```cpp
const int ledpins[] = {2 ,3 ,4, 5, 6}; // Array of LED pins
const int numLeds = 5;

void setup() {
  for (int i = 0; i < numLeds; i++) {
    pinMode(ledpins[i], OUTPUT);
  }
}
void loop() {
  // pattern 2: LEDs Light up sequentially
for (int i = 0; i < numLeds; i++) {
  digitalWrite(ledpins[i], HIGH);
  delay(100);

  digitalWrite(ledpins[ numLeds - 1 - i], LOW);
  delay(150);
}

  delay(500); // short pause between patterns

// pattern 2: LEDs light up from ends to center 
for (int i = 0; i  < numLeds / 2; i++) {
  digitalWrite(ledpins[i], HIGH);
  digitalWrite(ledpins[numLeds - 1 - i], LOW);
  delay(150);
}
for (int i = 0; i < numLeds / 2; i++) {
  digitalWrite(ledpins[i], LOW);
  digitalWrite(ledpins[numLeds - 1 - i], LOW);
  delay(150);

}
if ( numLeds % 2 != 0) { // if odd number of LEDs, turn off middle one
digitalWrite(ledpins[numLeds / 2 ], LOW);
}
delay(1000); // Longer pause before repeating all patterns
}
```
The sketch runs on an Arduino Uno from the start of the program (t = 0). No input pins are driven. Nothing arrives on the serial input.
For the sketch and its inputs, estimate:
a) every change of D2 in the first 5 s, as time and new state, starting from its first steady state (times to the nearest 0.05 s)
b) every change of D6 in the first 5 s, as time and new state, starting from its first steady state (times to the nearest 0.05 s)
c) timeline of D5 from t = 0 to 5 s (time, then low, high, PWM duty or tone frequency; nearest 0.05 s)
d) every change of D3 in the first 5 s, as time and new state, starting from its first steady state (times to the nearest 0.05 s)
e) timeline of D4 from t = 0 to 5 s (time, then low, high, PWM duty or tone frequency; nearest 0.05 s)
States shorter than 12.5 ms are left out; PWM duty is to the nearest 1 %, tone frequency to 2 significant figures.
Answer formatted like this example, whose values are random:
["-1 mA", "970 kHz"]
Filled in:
["0 s high; 1.1 s low; 1.75 s high; 2.05 s low; 3.35 s high; 4.45 s low", "0 s low; 1 s high; 1.75 s low; 4.35 s high", "0 s low; 0.75 s high; 1.9 s low; 4.1 s high", "0 s low; 0.25 s high; 0.85 s low; 1.9 s high; 2.2 s low; 3.6 s high; 4.2 s low", "0 s low; 0.5 s high; 0.6 s low; 3.85 s high; 3.95 s low"]
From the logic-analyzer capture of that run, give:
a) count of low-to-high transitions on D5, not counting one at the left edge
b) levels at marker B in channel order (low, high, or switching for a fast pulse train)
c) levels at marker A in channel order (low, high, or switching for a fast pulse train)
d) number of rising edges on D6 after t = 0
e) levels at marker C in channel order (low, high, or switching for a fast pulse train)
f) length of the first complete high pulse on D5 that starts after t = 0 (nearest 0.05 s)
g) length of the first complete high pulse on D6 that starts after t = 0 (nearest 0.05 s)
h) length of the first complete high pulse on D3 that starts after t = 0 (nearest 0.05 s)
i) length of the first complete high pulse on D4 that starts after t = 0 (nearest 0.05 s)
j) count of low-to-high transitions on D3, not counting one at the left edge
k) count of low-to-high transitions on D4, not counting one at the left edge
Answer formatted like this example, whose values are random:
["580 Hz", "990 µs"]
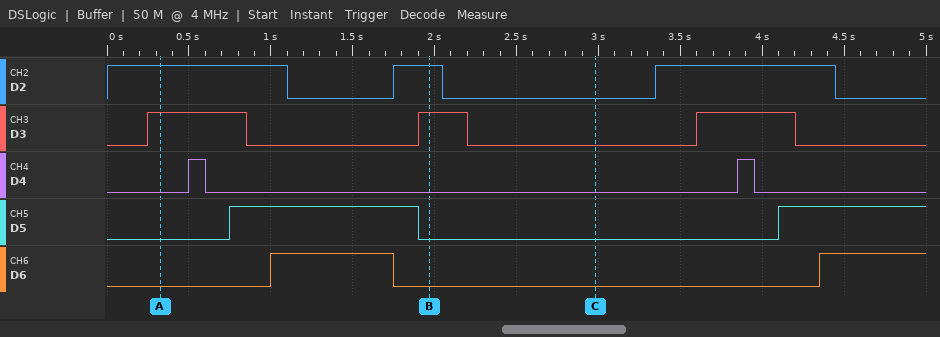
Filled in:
["2", "D2 high, D3 high, D4 low, D5 low, D6 low", "D2 high, D3 high, D4 low, D5 low, D6 low", "2", "D2 low, D3 low, D4 low, D5 low, D6 low", "1.15 s", "0.75 s", "0.60 s", "0.10 s", "3", "2"]
